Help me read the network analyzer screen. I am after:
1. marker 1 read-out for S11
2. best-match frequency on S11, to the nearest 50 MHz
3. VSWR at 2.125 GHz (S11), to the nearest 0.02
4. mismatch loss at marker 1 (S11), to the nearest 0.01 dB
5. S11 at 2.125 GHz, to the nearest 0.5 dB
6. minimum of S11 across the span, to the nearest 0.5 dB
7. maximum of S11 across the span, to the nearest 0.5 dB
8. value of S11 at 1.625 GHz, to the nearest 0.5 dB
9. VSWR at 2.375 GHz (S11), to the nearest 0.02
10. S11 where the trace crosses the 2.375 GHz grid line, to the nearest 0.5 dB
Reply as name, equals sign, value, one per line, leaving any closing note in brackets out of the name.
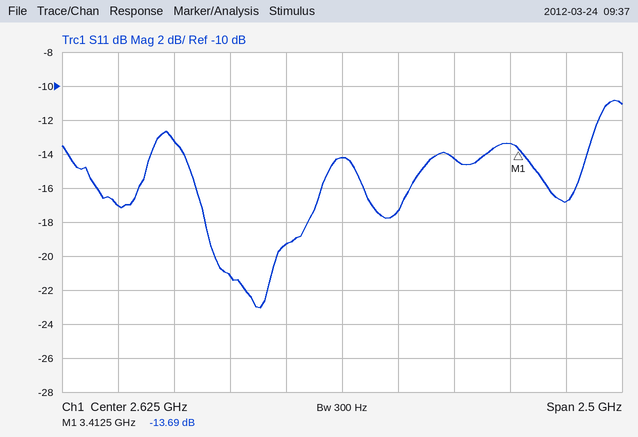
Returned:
marker 1 read-out for S11 = -13.69 dB
best-match frequency on S11, to the nearest 50 MHz = 2.25 GHz
VSWR at 2.125 GHz (S11), to the nearest 0.02 = 1.20
mismatch loss at marker 1 (S11), to the nearest 0.01 dB = 0.19 dB
S11 at 2.125 GHz, to the nearest 0.5 dB = -21.0 dB
minimum of S11 across the span, to the nearest 0.5 dB = -23.0 dB
maximum of S11 across the span, to the nearest 0.5 dB = -11.0 dB
value of S11 at 1.625 GHz, to the nearest 0.5 dB = -17.0 dB
VSWR at 2.375 GHz (S11), to the nearest 0.02 = 1.24
S11 where the trace crosses the 2.375 GHz grid line, to the nearest 0.5 dB = -19.5 dB
